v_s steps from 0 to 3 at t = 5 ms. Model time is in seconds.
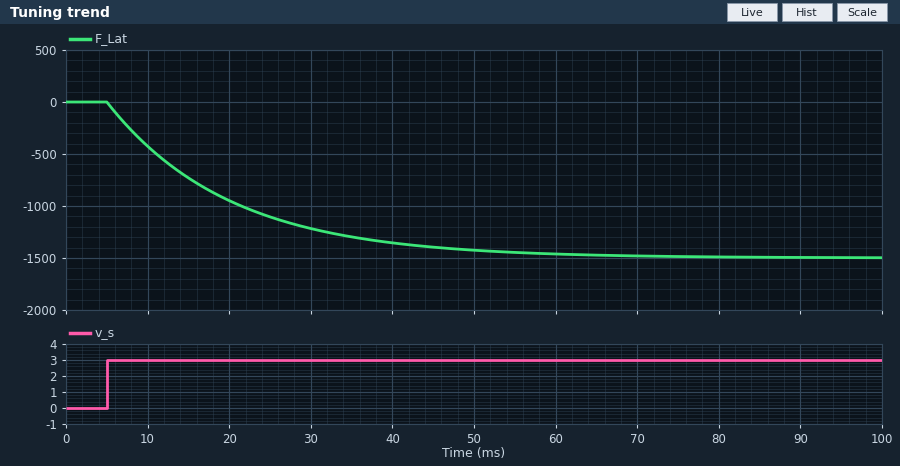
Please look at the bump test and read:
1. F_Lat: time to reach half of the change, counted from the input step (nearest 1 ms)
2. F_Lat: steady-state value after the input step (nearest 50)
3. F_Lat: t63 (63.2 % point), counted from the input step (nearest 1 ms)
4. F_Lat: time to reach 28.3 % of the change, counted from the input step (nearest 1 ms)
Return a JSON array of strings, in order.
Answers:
["10 ms", "-1500", "15 ms", "5 ms"]
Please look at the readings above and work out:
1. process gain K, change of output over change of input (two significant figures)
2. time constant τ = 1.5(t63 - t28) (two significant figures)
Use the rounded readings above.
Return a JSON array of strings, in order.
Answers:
["-500", "15 ms"]
